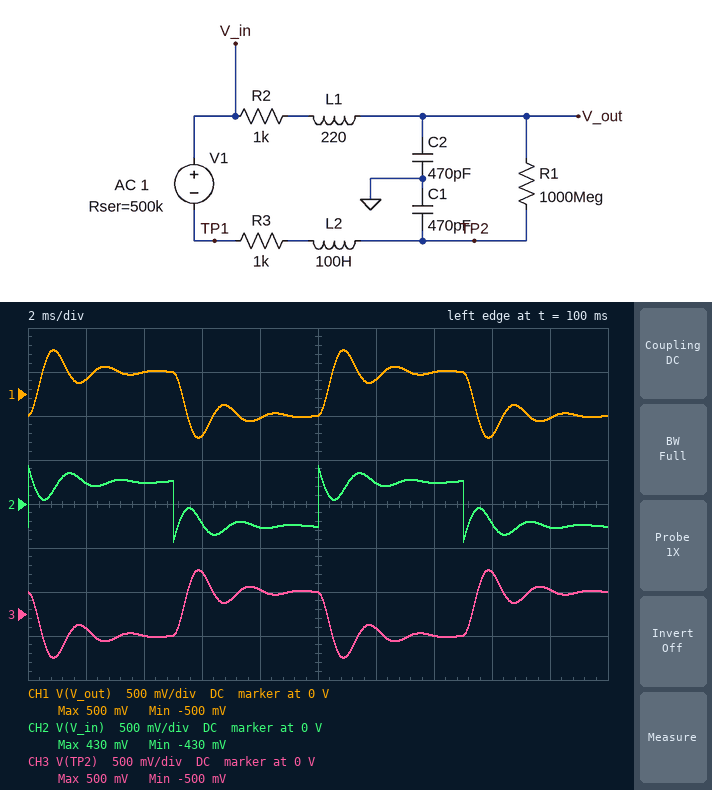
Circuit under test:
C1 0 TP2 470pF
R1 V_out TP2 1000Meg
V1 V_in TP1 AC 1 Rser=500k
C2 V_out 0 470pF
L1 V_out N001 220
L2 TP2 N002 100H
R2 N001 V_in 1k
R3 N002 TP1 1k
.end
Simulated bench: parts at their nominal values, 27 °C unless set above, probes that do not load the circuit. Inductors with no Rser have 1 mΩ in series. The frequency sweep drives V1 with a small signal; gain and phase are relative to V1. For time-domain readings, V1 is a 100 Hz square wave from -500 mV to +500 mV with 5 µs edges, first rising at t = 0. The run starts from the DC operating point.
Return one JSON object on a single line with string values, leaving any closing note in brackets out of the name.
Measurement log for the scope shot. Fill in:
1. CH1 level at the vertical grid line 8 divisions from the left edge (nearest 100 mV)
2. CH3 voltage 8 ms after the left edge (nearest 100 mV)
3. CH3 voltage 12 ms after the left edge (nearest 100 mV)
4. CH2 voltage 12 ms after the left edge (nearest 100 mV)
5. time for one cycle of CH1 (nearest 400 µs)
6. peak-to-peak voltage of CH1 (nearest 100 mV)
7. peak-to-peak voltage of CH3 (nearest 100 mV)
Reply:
{"CH1 level at the vertical grid line 8 divisions from the left edge": "-500 mV", "CH3 voltage 8 ms after the left edge": "300 mV", "CH3 voltage 12 ms after the left edge": "-200 mV", "CH2 voltage 12 ms after the left edge": "200 mV", "time for one cycle of CH1": "10.0 ms", "peak-to-peak voltage of CH1": "1.0 V", "peak-to-peak voltage of CH3": "1.0 V"}
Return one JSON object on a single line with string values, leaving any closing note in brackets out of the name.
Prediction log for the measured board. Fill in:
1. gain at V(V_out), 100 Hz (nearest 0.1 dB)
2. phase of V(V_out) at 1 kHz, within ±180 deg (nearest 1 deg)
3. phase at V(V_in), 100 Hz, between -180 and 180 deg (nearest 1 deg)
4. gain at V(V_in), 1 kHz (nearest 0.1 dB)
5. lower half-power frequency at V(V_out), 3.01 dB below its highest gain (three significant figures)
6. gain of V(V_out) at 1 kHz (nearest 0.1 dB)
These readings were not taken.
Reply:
{"gain at V(V_out), 100 Hz": "-5.8 dB", "phase of V(V_out) at 1 kHz, within ±180 deg": "-159 deg", "phase at V(V_in), 100 Hz, between -180 and 180 deg": "-4 deg", "gain at V(V_in), 1 kHz": "-2.7 dB", "lower half-power frequency at V(V_out), 3.01 dB below its highest gain": "405 Hz", "gain of V(V_out) at 1 kHz": "-12.5 dB"}
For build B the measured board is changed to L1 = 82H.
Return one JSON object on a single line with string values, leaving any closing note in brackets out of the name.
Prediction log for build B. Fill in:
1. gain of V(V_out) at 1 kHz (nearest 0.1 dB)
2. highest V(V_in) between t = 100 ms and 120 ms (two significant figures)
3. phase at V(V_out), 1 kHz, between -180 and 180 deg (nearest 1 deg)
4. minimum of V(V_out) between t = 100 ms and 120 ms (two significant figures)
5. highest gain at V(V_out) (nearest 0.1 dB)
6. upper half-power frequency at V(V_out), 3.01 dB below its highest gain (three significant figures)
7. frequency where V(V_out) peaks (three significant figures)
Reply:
{"gain of V(V_out) at 1 kHz": "-6.1 dB", "highest V(V_in) between t = 100 ms and 120 ms": "330 mV", "phase at V(V_out), 1 kHz, between -180 and 180 deg": "-133 deg", "minimum of V(V_out) between t = 100 ms and 120 ms": "-450 mV", "highest gain at V(V_out)": "-0.8 dB", "upper half-power frequency at V(V_out), 3.01 dB below its highest gain": "906 Hz", "frequency where V(V_out) peaks": "704 Hz"}
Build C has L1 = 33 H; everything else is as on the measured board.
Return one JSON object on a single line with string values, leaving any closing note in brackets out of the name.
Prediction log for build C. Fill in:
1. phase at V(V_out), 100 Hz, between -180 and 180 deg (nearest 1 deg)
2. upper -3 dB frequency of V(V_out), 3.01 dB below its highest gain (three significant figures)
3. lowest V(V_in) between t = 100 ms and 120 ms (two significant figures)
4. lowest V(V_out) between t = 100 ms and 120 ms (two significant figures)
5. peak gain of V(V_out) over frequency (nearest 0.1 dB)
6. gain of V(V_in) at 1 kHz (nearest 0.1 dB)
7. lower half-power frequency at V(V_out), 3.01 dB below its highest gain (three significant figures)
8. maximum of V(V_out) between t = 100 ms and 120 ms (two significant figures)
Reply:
{"phase at V(V_out), 100 Hz, between -180 and 180 deg": "-4 deg", "upper -3 dB frequency of V(V_out), 3.01 dB below its highest gain": "1.07 kHz", "lowest V(V_in) between t = 100 ms and 120 ms": "-350 mV", "lowest V(V_out) between t = 100 ms and 120 ms": "-410 mV", "peak gain of V(V_out) over frequency": "-2.0 dB", "gain of V(V_in) at 1 kHz": "-12.1 dB", "lower half-power frequency at V(V_out), 3.01 dB below its highest gain": "346 Hz", "maximum of V(V_out) between t = 100 ms and 120 ms": "410 mV"}
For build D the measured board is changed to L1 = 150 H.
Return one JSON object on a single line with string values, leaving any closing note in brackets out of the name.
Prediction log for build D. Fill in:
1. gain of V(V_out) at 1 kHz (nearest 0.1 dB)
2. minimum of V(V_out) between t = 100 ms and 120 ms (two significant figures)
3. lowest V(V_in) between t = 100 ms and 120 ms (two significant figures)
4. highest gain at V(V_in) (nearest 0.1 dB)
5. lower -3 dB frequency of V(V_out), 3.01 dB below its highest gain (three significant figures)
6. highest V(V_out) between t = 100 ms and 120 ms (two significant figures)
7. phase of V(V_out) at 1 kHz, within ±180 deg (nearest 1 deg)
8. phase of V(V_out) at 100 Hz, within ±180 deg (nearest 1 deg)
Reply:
{"gain of V(V_out) at 1 kHz": "-9.6 dB", "minimum of V(V_out) between t = 100 ms and 120 ms": "-480 mV", "lowest V(V_in) between t = 100 ms and 120 ms": "-350 mV", "highest gain at V(V_in)": "-4.4 dB", "lower -3 dB frequency of V(V_out), 3.01 dB below its highest gain": "420 Hz", "highest V(V_out) between t = 100 ms and 120 ms": "480 mV", "phase of V(V_out) at 1 kHz, within ±180 deg": "-151 deg", "phase of V(V_out) at 100 Hz, within ±180 deg": "-4 deg"}
